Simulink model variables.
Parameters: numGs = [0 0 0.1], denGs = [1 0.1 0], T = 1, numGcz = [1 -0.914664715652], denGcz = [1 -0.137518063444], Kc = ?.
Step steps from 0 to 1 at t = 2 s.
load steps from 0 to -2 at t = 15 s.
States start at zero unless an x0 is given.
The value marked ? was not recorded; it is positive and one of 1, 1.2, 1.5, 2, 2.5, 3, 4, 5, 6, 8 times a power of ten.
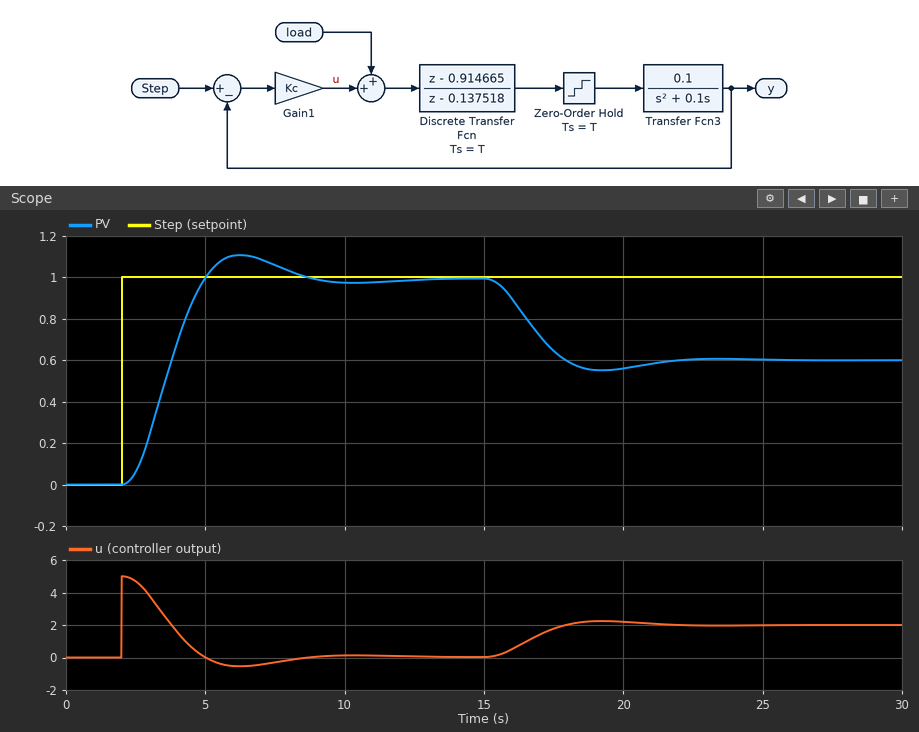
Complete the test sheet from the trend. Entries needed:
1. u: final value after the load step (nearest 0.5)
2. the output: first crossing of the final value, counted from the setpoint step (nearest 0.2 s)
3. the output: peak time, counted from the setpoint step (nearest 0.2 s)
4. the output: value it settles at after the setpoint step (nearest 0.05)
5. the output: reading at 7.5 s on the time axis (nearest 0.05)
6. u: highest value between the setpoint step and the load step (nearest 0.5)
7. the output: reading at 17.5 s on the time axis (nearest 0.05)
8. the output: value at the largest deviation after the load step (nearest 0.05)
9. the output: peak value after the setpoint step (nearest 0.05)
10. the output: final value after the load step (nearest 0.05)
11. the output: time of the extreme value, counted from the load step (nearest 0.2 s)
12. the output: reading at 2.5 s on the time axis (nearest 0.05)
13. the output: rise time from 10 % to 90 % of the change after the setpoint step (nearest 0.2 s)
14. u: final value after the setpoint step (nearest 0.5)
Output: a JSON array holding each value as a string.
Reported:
["2.0", "3.0 s", "4.2 s", "1.00", "1.05", "5.0", "0.65", "0.55", "1.10", "0.60", "4.2 s", "0.05", "2.0 s", "0.0"]
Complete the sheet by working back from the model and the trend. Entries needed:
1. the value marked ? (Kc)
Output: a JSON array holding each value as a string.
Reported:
["5"]
